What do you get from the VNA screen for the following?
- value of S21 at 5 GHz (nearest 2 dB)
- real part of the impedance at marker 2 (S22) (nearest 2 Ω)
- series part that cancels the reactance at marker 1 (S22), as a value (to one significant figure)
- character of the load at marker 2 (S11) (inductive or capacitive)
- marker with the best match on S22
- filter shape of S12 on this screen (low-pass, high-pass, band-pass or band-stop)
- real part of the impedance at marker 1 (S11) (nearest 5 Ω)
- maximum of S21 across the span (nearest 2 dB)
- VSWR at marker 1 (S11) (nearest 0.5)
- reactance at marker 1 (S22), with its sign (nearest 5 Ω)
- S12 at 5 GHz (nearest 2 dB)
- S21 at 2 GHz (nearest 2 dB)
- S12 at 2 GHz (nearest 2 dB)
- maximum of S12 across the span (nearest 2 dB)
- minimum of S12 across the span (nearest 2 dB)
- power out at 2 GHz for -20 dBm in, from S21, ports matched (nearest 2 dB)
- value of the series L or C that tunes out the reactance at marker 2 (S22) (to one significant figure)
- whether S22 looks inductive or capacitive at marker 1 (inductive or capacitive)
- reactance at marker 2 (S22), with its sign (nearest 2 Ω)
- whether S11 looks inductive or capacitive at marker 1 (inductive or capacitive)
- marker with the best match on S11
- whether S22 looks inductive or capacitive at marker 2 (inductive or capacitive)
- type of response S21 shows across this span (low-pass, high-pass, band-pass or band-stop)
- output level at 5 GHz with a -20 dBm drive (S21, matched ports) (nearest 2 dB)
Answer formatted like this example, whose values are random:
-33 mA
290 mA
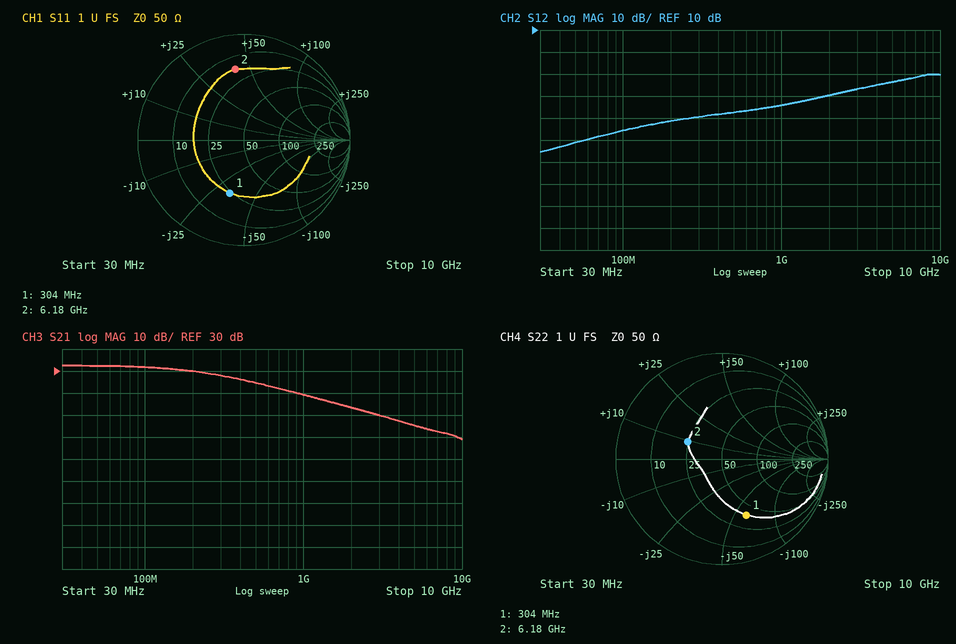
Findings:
6 dB
24 Ω
30 nH
inductive
marker 2
high-pass
25 Ω
32 dB
3.0
-60 Ω
-14 dB
14 dB
-20 dB
-10 dB
-46 dB
-6 dBm
3 pF
capacitive
+10 Ω
capacitive
marker 1
inductive
low-pass
-14 dBm
